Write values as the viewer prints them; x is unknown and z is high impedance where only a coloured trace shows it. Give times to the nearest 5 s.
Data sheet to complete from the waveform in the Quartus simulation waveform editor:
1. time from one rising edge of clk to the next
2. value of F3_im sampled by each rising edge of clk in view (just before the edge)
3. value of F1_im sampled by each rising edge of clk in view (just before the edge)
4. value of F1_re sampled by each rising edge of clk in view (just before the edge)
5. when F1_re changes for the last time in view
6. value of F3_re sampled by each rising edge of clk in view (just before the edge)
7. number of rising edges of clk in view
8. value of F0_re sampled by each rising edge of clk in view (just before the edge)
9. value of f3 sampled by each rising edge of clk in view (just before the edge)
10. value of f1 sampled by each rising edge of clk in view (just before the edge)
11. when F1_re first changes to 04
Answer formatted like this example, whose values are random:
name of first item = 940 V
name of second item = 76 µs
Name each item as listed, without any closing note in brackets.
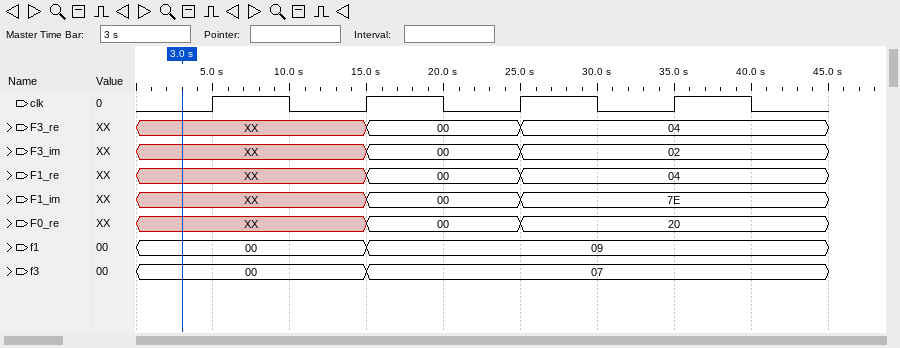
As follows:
time from one rising edge of clk to the next = 10 s
value of F3_im sampled by each rising edge of clk in view = XX, XX, 00, 02
value of F1_im sampled by each rising edge of clk in view = XX, XX, 00, 7E
value of F1_re sampled by each rising edge of clk in view = XX, XX, 00, 04
when F1_re changes for the last time in view = 25 s
value of F3_re sampled by each rising edge of clk in view = XX, XX, 00, 04
number of rising edges of clk in view = 4
value of F0_re sampled by each rising edge of clk in view = XX, XX, 00, 20
value of f3 sampled by each rising edge of clk in view = 00, 00, 07, 07
value of f1 sampled by each rising edge of clk in view = 00, 00, 09, 09
when F1_re first changes to 04 = 25 s
